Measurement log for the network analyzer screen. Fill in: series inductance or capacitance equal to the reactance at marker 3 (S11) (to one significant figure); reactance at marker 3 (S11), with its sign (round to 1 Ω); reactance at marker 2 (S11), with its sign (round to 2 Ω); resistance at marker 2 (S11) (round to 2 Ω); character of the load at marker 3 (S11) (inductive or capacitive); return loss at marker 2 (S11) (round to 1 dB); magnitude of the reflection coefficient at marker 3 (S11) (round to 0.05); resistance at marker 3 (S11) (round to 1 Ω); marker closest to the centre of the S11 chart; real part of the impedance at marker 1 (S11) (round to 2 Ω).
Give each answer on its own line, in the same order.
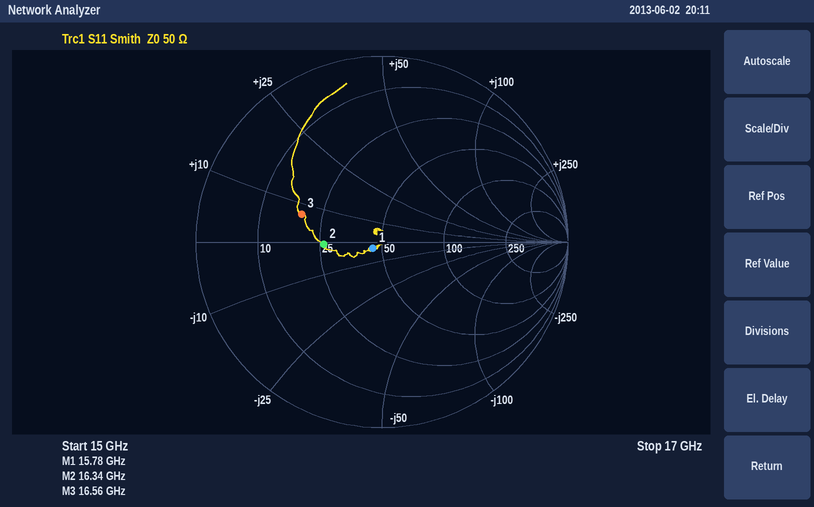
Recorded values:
70 pH
+7 Ω
0 Ω
26 Ω
inductive
10 dB
0.45
19 Ω
marker 1
46 Ω
